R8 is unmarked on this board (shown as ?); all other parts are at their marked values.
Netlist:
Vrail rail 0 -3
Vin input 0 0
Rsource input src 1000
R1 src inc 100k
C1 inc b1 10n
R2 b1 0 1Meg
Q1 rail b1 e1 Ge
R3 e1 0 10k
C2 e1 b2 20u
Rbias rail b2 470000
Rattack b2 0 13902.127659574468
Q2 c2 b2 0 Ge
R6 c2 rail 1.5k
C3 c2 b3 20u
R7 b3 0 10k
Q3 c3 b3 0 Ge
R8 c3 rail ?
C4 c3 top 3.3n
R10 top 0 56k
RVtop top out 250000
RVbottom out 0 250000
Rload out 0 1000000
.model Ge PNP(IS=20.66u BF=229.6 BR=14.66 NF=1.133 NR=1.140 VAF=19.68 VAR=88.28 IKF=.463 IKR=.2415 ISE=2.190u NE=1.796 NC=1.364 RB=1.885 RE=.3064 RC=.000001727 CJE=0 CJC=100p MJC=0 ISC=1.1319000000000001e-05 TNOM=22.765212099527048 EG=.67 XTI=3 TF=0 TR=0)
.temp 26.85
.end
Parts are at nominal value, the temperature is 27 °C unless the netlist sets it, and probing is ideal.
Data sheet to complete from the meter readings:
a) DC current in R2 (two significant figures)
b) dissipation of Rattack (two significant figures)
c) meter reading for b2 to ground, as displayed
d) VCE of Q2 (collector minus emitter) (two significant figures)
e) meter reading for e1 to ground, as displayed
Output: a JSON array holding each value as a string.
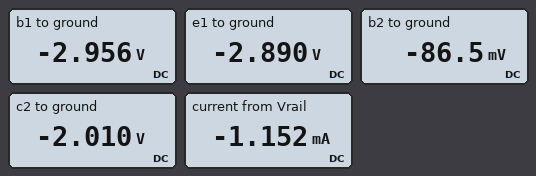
["3.0 µA", "540 nW", "-86.5 mV", "-2.0 V", "-2.890 V"]
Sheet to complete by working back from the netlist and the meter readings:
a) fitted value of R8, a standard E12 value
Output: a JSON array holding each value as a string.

["15 kΩ"]
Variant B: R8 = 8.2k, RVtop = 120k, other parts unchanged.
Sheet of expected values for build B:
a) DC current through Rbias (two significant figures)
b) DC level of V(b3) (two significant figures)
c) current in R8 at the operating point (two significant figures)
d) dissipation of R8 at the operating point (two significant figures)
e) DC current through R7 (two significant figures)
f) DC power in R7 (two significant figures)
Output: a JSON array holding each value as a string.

["6.2 µA", "-68 mV", "330 µA", "910 µW", "6.8 µA", "460 nW"]
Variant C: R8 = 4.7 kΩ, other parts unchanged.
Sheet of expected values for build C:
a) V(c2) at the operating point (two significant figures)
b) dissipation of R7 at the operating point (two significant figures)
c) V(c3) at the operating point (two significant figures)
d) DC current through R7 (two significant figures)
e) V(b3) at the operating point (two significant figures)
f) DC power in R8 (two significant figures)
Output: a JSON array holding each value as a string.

["-2.0 V", "470 nW", "-1.3 V", "6.8 µA", "-68 mV", "590 µW"]
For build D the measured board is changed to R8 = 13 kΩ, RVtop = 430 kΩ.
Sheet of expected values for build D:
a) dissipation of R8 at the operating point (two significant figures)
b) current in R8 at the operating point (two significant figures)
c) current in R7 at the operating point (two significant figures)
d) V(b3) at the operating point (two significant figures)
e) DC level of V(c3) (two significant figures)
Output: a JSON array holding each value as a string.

["640 µW", "220 µA", "5.7 µA", "-57 mV", "-110 mV"]
